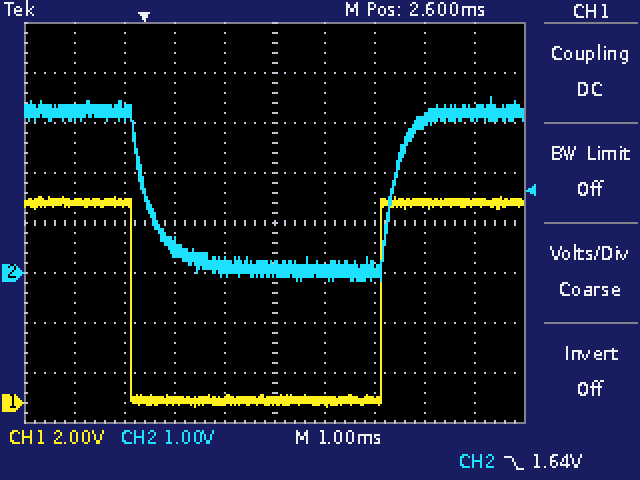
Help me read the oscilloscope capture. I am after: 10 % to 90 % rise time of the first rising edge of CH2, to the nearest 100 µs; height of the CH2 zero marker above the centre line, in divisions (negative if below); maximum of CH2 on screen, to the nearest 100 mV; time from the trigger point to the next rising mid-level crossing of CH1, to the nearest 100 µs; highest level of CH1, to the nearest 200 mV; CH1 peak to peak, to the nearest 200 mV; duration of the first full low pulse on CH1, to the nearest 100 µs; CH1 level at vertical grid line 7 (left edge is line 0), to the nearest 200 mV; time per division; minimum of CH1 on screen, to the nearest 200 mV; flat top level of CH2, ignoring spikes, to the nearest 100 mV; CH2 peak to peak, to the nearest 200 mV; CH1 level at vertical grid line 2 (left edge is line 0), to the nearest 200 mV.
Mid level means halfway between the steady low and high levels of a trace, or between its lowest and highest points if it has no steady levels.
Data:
600 µs
-1.0 div
3.5 V
4.7 ms
8.2 V
8.4 V
5.0 ms
200 mV
1 ms
-200 mV
3.2 V
3.6 V
8.0 V
